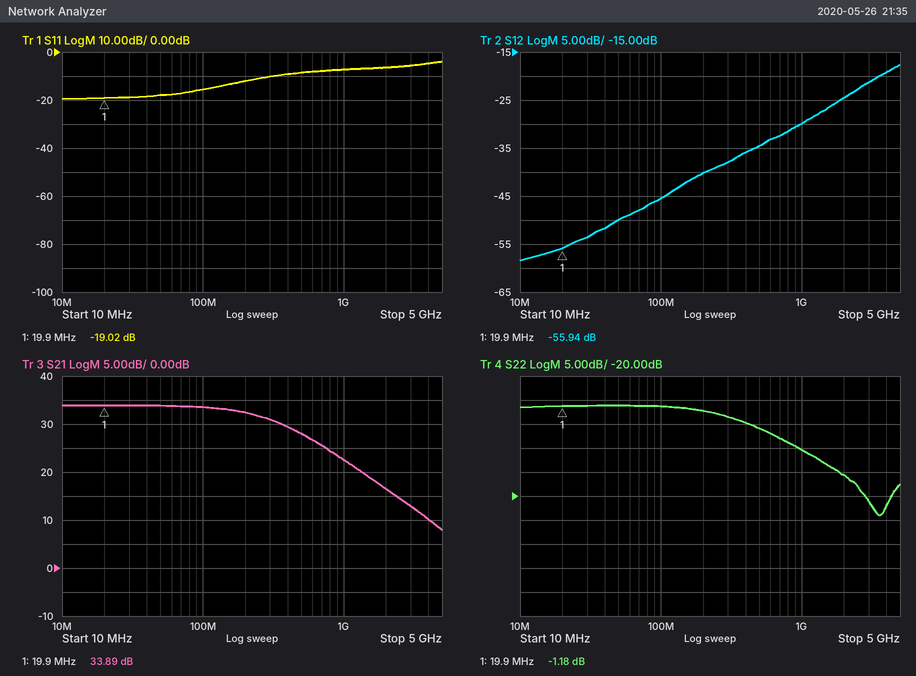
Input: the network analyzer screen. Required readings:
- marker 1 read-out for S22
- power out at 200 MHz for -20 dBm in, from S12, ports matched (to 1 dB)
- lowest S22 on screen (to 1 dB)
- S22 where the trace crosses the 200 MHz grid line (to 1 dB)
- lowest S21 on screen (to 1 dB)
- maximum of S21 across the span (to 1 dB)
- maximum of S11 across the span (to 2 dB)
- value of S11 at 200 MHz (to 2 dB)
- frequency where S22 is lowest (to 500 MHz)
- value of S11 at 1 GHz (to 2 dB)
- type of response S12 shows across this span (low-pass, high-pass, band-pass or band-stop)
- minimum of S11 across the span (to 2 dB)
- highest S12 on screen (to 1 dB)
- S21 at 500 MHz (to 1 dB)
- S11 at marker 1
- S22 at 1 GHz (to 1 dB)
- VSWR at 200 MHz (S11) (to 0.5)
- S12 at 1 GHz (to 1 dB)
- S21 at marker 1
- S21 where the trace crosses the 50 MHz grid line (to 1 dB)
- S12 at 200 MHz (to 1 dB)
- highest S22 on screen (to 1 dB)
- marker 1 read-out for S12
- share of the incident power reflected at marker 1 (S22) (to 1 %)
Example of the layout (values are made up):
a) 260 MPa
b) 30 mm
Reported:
a) -1.18 dB
b) -60 dBm
c) -24 dB
d) -2 dB
e) 8 dB
f) 34 dB
g) -4 dB
h) -12 dB
i) 3.5 GHz
j) -8 dB
k) high-pass
l) -20 dB
m) -18 dB
n) 28 dB
o) -19.02 dB
p) -10 dB
q) 1.5
r) -30 dB
s) 33.89 dB
t) 34 dB
u) -40 dB
v) -1 dB
w) -55.94 dB
x) 76 %
